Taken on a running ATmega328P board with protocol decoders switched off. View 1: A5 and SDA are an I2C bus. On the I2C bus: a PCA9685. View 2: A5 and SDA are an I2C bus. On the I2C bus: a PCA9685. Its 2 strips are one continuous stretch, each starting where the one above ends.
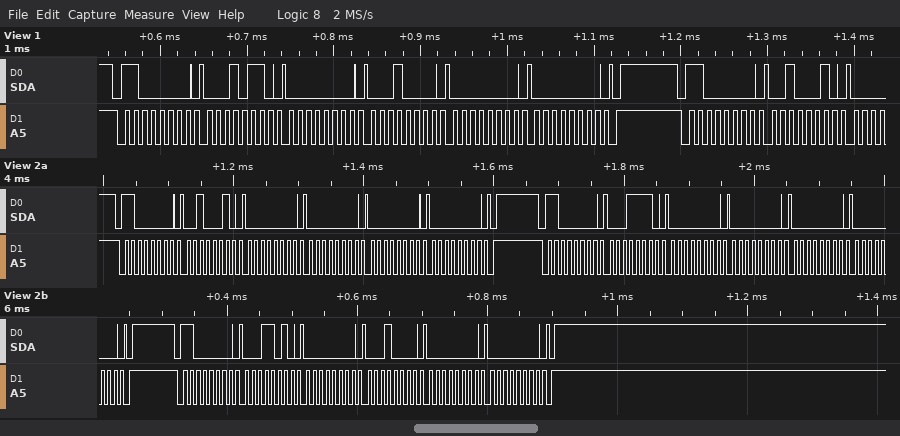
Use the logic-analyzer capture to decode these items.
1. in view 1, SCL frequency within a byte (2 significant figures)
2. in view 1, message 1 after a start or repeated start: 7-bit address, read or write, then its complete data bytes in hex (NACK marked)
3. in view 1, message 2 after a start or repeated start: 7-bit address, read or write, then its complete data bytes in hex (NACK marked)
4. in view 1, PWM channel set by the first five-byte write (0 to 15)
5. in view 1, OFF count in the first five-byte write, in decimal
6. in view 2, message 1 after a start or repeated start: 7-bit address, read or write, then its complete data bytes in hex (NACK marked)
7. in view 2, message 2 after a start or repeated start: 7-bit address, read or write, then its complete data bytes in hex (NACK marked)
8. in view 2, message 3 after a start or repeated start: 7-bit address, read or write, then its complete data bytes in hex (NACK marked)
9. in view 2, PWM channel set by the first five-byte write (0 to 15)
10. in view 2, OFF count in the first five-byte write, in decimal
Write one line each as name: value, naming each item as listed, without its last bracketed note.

in view 1, SCL frequency within a byte: 100 kHz
in view 1, message 1 after a start or repeated start: 7-bit address, read or write, then its complete data bytes in hex: 0x60 write: 16 00 10 00 00
in view 1, message 2 after a start or repeated start: 7-bit address, read or write, then its complete data bytes in hex: 0x60 write: 22
in view 1, PWM channel set by the first five-byte write: 4
in view 1, OFF count in the first five-byte write, in decimal: 0
in view 2, message 1 after a start or repeated start: 7-bit address, read or write, then its complete data bytes in hex: 0x60 write: 22 00 00 00 00
in view 2, message 2 after a start or repeated start: 7-bit address, read or write, then its complete data bytes in hex: 0x60 write: 1E 00 00 00 00
in view 2, message 3 after a start or repeated start: 7-bit address, read or write, then its complete data bytes in hex: 0x60 write: 1A 00 10 00 00
in view 2, PWM channel set by the first five-byte write: 7
in view 2, OFF count in the first five-byte write, in decimal: 0
